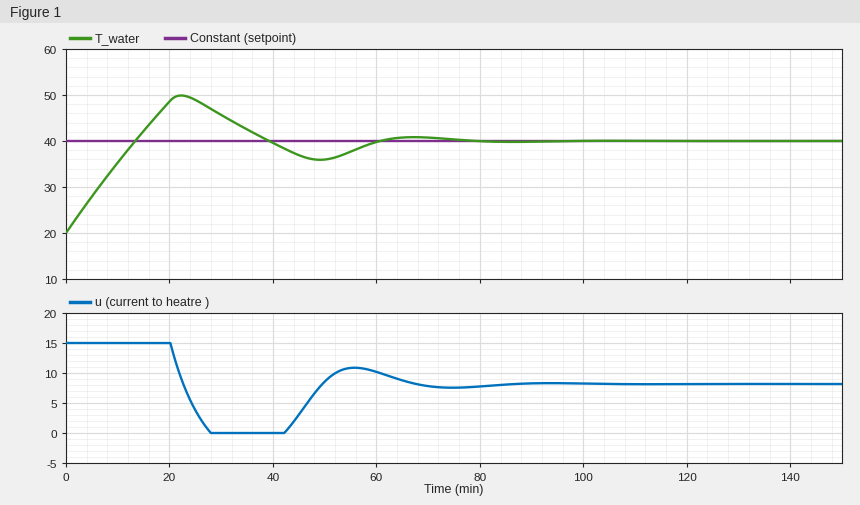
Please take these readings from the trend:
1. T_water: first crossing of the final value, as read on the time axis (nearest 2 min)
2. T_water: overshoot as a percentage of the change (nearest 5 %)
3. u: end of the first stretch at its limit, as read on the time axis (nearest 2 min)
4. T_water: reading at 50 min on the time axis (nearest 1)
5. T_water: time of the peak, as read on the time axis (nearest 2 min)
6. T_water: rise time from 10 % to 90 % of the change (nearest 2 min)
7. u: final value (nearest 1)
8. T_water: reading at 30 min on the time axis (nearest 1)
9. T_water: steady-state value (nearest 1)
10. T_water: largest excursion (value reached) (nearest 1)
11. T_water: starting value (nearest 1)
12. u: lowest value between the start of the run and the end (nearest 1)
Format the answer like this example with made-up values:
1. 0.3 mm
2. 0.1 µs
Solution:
1. 14 min
2. 50 %
3. 20 min
4. 36
5. 22 min
6. 10 min
7. 8
8. 46
9. 40
10. 50
11. 20
12. 0
